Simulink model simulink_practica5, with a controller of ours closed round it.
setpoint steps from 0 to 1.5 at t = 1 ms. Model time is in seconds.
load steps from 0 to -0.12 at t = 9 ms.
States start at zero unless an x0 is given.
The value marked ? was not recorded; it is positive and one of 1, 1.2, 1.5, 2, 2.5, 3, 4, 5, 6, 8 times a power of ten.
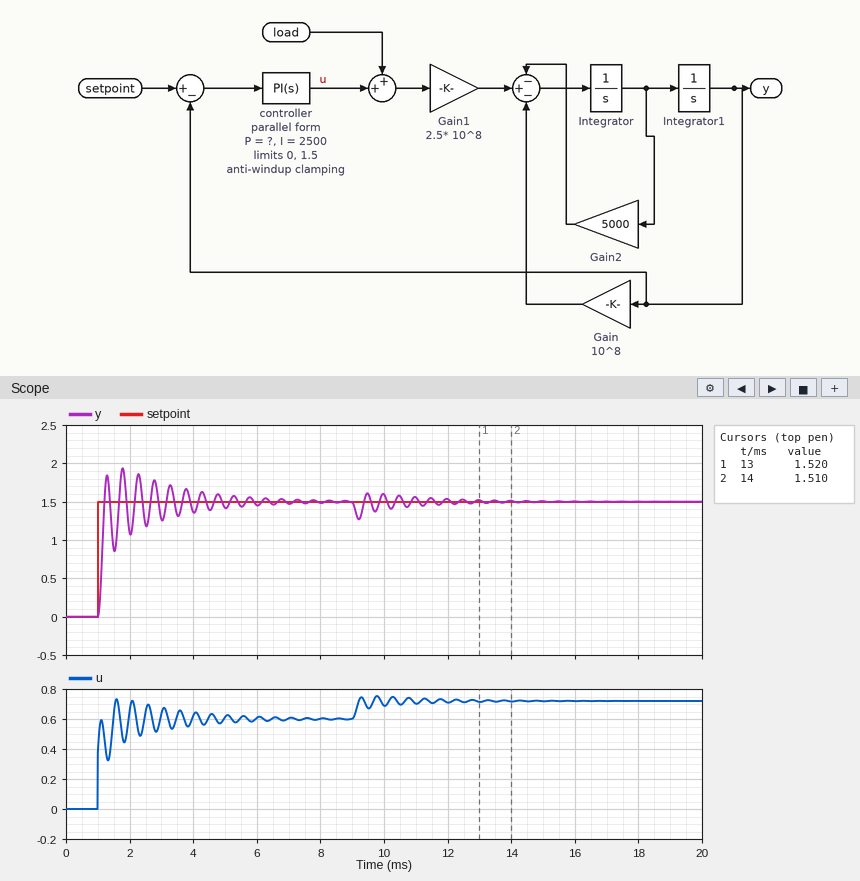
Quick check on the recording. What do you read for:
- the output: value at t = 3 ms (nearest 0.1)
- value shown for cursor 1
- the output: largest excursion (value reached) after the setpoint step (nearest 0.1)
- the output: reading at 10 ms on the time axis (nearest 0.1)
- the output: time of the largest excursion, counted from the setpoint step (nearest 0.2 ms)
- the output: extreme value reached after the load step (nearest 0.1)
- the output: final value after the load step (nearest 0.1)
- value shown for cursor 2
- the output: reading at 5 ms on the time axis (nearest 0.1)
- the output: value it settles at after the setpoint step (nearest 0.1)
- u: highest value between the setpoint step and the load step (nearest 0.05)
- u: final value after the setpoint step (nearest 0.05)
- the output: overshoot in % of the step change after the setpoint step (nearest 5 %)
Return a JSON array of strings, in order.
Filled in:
["1.3", "1.520", "1.9", "1.6", "0.8 ms", "1.3", "1.5", "1.510", "1.4", "1.5", "0.75", "0.60", "30 %"]
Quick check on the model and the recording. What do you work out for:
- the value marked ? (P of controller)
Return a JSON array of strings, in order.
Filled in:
["0.25"]
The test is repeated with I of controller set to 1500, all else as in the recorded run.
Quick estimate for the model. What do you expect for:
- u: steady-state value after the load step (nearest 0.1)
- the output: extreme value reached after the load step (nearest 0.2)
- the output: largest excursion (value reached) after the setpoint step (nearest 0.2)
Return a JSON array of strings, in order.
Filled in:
["0.7", "1.2", "1.6"]
